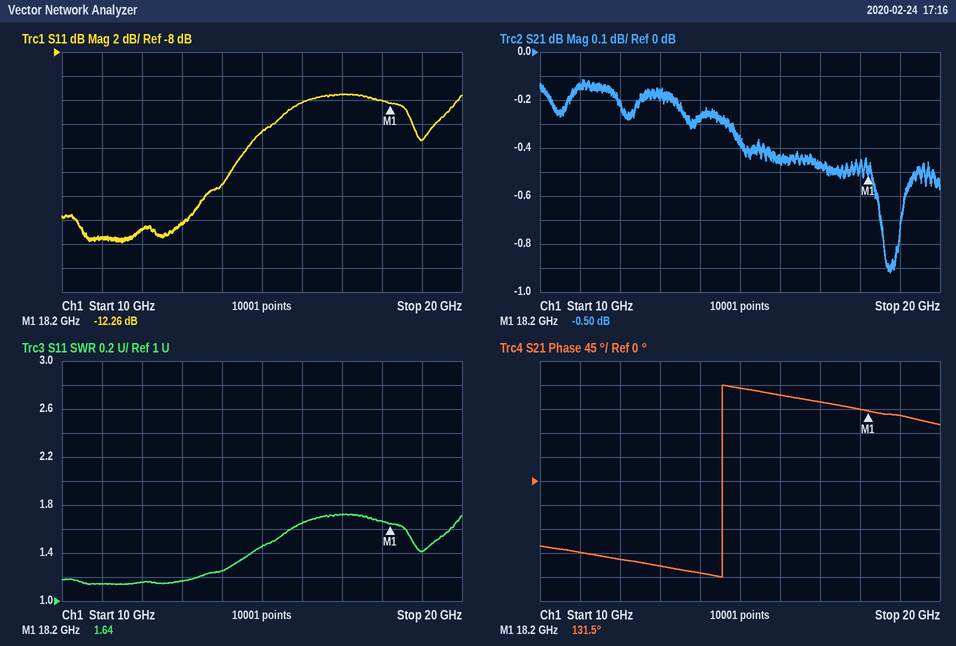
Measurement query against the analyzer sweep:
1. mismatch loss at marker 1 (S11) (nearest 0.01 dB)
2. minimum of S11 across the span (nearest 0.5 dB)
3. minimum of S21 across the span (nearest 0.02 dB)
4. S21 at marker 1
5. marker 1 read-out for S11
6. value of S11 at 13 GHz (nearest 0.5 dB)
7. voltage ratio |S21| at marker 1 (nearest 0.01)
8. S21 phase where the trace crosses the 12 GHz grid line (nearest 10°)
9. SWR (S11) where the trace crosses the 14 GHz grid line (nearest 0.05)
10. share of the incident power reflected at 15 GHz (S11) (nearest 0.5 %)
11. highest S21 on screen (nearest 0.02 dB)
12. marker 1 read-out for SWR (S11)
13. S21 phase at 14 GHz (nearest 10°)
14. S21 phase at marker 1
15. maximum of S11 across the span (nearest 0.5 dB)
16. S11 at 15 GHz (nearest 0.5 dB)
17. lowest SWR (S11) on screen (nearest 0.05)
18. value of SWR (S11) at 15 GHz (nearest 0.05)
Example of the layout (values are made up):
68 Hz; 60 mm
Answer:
0.27 dB; -24.0 dB; -0.92 dB; -0.50 dB; -12.26 dB; -22.5 dB; 0.94; -150°; 1.25; 3.5 %; -0.12 dB; 1.64; -170°; 131.5°; -11.5 dB; -14.5 dB; 1.15; 1.45
